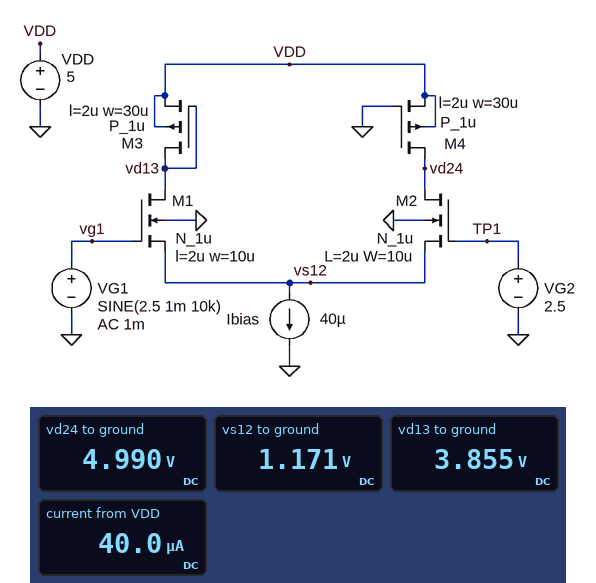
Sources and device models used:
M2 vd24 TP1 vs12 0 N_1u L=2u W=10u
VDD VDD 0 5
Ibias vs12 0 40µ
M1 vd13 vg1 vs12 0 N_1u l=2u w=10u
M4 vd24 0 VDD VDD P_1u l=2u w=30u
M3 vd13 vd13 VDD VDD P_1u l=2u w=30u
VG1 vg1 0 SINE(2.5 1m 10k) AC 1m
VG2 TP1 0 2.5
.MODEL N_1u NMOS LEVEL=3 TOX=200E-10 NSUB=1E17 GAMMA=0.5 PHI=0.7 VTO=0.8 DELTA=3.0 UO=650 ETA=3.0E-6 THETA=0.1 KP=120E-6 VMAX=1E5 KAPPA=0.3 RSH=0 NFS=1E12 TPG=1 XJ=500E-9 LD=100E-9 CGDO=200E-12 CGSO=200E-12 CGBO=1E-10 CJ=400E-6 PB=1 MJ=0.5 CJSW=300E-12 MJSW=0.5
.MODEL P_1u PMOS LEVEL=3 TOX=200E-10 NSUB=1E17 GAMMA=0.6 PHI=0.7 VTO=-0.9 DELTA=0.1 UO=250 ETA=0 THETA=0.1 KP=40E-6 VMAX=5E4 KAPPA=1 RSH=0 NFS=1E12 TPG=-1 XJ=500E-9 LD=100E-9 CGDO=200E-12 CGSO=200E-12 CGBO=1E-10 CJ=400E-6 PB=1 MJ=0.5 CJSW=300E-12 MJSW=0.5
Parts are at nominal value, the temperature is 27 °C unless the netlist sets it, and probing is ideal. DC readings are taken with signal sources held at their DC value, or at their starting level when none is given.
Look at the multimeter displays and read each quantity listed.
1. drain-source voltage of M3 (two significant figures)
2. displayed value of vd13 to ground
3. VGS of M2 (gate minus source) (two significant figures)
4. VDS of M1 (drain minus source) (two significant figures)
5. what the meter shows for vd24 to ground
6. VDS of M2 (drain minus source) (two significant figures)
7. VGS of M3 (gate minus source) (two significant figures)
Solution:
-1.1 V
3.855 V
1.3 V
2.7 V
4.990 V
3.8 V
-1.1 V
